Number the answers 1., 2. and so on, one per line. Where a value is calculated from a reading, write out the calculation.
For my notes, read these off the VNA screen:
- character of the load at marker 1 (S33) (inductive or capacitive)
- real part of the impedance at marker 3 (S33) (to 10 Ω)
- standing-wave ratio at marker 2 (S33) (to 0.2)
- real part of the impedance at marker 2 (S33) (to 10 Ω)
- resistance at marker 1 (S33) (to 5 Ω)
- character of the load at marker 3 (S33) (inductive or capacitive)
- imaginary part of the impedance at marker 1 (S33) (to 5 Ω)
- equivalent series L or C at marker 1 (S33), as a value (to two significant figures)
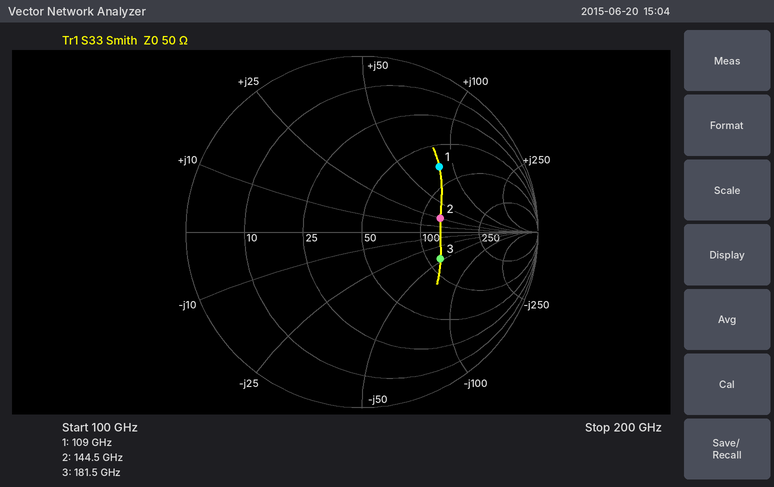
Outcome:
1. inductive
2. 120 Ω
3. 2.6
4. 130 Ω
5. 75 Ω
6. capacitive
7. +80 Ω
8. L = 80 Ω/(2π × 109 GHz) ≈ 117 pH, so 120 pH to two significant figures
